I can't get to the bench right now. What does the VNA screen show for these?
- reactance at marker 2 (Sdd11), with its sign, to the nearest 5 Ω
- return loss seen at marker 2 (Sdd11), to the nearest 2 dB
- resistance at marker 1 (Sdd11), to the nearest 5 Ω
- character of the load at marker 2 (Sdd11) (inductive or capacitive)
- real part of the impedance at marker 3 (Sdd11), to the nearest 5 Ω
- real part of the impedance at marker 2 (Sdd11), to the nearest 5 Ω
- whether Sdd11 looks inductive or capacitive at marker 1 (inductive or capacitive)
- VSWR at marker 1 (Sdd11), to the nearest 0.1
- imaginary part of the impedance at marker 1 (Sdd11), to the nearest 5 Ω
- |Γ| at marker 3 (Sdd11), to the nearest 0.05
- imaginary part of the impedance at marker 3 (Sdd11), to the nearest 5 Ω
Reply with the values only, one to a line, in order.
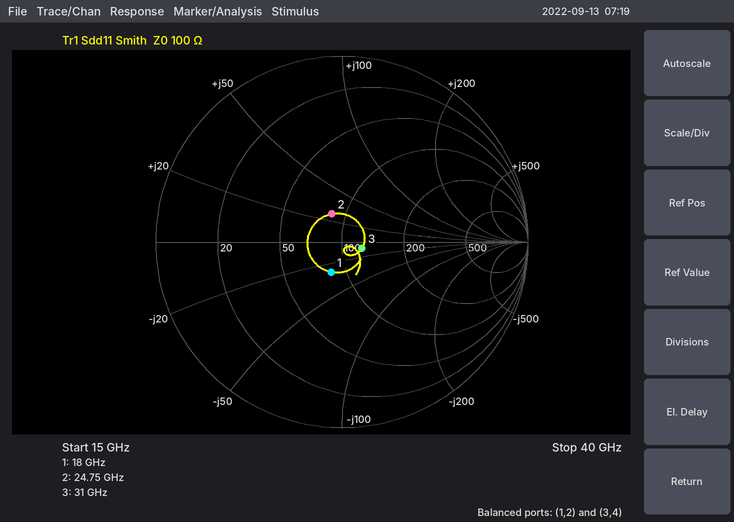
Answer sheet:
+25 Ω
16 dB
85 Ω
inductive
125 Ω
85 Ω
capacitive
1.4
-30 Ω
0.10
-10 Ω
